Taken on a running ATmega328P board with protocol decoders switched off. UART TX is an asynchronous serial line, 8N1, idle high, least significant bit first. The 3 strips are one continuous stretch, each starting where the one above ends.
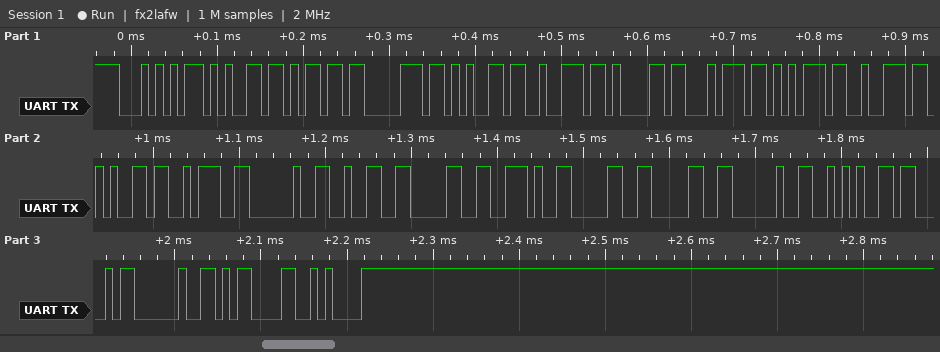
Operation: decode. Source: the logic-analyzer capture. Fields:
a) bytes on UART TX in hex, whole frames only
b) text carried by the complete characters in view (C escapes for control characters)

54 65 6D 70 65 72 61 74 75 72 65 3A 20 32 30 2E 30 30 20 2A 43 20 0D 0A
"Temperature: 20.00 *C \r\n"
